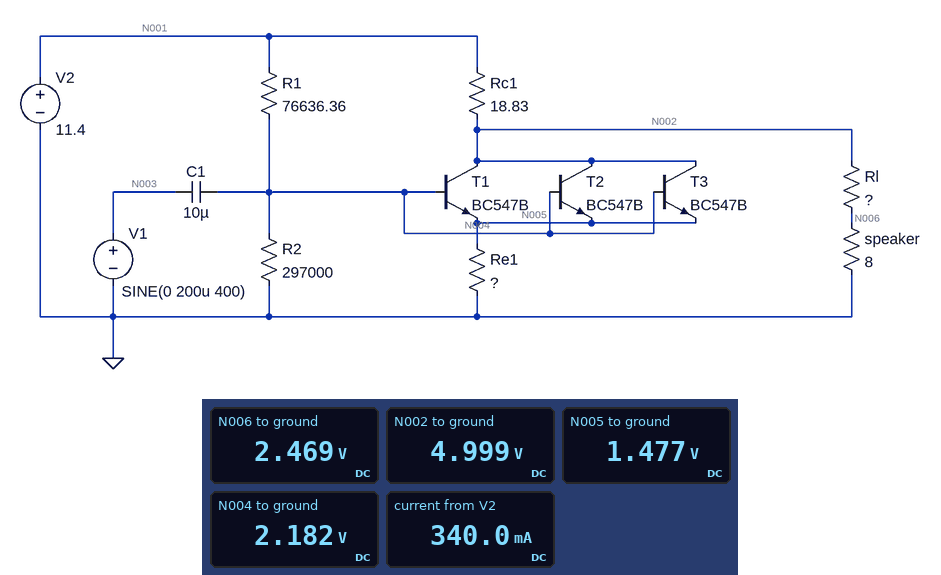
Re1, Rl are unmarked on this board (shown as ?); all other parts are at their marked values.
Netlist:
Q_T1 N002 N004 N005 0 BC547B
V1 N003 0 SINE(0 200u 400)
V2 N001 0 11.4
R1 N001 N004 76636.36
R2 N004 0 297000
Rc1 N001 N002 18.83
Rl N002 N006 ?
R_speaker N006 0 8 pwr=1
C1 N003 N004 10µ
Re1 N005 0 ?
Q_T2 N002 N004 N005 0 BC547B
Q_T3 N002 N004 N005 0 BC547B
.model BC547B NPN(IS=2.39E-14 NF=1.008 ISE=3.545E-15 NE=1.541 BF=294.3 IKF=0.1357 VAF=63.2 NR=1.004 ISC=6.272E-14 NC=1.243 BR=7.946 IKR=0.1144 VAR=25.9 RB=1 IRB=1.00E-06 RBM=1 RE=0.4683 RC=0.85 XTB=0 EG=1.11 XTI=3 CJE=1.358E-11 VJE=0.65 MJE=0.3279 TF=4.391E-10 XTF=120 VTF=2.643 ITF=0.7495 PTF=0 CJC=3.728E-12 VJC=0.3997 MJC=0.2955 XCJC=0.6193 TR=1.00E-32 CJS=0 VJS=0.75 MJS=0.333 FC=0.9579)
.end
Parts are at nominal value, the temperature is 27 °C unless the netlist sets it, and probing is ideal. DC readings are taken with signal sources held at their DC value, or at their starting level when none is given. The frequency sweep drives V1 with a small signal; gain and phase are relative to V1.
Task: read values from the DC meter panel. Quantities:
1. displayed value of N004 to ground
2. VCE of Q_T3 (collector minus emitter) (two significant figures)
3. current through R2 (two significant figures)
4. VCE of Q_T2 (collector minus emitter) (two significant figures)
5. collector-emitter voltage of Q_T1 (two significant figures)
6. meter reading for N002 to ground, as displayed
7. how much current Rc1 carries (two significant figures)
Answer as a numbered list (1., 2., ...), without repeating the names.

1. 2.182 V
2. 3.5 V
3. 7.3 µA
4. 3.5 V
5. 3.5 V
6. 4.999 V
7. 340 mA
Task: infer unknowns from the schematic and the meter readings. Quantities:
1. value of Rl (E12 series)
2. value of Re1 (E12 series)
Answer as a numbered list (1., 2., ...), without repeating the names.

1. 8.2 Ω
2. 47 Ω
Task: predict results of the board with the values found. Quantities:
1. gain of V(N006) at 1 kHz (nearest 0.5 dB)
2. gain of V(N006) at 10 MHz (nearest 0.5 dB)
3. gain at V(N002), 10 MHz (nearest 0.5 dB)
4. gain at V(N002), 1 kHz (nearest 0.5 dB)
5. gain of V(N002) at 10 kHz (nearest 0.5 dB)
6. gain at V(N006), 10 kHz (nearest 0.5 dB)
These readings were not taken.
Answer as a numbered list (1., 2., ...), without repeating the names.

1. -21.0 dB
2. -21.0 dB
3. -15.0 dB
4. -15.0 dB
5. -15.0 dB
6. -21.0 dB
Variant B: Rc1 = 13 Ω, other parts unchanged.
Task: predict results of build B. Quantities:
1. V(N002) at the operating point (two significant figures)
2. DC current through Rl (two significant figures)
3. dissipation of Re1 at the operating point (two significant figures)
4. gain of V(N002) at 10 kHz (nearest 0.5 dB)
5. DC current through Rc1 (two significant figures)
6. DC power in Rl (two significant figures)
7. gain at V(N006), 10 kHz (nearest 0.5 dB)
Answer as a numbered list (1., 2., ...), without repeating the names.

1. 6.1 V
2. 380 mA
3. 48 mW
4. -16.5 dB
5. 410 mA
6. 1.2 W
7. -22.5 dB
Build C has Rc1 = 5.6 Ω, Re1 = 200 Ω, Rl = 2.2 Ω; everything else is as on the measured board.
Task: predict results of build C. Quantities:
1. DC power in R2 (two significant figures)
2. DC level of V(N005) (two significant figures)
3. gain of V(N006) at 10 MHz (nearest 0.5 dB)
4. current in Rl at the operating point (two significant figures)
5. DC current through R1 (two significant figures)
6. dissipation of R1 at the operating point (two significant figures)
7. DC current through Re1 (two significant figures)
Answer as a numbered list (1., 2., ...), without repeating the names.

1. 75 µW
2. 4.0 V
3. -37.0 dB
4. 710 mA
5. 87 µA
6. 580 µW
7. 20 mA
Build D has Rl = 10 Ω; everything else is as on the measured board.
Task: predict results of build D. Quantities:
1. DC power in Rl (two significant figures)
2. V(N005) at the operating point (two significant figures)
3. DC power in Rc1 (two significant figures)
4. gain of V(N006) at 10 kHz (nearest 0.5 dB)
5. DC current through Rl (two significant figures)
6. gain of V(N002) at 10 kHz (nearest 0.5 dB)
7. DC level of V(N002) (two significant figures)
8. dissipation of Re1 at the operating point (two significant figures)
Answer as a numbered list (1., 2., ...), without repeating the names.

1. 860 mW
2. 1.5 V
3. 2.0 W
4. -21.5 dB
5. 290 mA
6. -14.5 dB
7. 5.3 V
8. 47 mW
